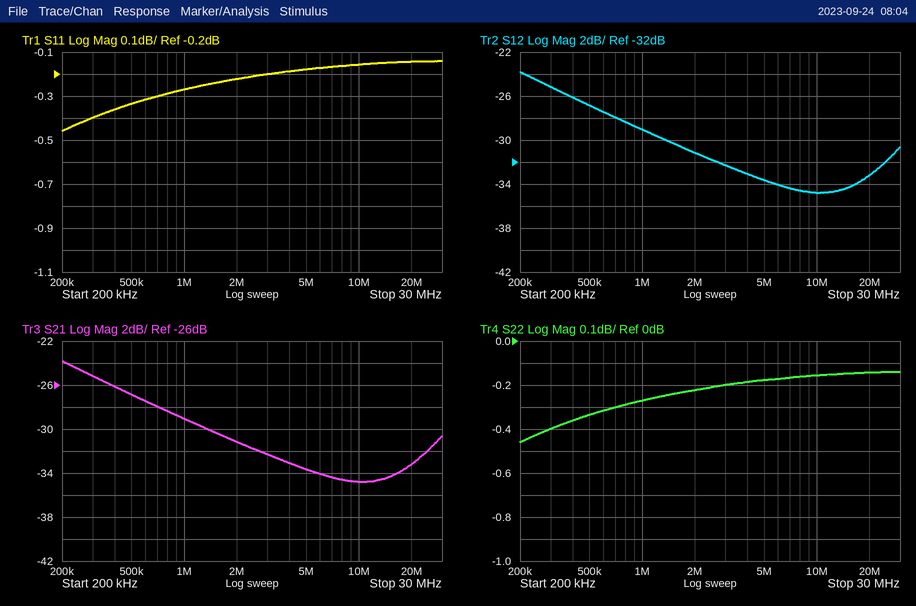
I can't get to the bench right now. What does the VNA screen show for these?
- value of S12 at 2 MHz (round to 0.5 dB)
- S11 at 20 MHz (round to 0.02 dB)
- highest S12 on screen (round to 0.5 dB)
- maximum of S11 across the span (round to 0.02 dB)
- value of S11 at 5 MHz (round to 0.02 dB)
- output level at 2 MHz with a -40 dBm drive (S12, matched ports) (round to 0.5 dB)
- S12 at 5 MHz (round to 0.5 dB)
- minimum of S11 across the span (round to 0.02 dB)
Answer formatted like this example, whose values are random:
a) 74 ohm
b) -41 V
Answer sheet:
a) -31.0 dB
b) -0.14 dB
c) -24.0 dB
d) -0.14 dB
e) -0.18 dB
f) -71.0 dBm
g) -33.5 dB
h) -0.46 dB
